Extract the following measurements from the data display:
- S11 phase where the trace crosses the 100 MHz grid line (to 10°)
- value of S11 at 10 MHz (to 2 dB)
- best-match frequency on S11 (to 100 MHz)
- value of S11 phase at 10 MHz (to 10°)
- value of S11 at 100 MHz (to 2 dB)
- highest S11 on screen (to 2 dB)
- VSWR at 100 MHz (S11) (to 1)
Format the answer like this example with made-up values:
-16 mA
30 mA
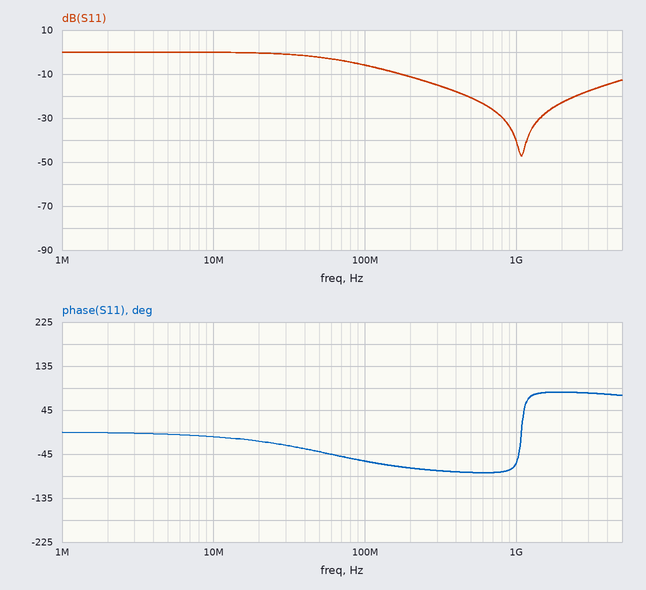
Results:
-60°
0 dB
1.1 GHz
-10°
-6 dB
0 dB
3
